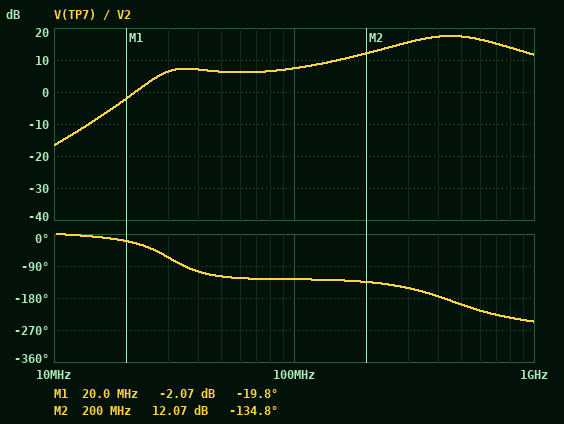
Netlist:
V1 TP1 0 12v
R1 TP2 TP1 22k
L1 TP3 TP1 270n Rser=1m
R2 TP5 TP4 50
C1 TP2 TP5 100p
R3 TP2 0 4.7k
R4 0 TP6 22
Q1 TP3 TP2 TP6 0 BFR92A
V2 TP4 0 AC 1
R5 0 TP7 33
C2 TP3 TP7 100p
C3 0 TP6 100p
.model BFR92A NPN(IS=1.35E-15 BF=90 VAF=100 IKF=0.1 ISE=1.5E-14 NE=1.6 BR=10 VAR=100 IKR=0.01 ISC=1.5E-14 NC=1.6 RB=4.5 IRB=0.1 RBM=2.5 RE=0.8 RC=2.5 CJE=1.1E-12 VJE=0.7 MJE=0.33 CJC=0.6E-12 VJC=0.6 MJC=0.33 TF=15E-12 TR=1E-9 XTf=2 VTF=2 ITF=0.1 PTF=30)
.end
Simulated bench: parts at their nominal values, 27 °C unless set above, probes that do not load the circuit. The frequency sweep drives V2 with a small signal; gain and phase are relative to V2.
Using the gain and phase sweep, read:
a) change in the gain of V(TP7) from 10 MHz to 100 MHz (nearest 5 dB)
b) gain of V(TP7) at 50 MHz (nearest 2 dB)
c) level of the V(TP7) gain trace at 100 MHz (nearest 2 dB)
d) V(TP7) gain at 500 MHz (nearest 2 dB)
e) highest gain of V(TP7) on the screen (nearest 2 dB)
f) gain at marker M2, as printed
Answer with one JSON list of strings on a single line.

["25 dB", "6 dB", "8 dB", "18 dB", "18 dB", "12.07 dB"]
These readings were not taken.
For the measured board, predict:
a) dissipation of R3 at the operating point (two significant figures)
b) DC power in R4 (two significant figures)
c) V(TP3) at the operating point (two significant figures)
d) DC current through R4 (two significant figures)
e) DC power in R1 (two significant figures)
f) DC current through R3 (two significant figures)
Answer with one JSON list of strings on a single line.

["320 µW", "8.2 mW", "12 V", "19 mA", "5.3 mW", "260 µA"]
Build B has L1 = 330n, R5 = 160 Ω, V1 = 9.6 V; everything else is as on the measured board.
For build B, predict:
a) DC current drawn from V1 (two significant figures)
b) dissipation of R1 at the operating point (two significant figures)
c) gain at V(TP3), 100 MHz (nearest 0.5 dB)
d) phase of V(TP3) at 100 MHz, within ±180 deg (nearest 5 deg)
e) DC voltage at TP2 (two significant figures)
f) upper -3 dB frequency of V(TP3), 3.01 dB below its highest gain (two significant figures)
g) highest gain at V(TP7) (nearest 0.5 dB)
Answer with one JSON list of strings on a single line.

["14 mA", "3.3 mW", "19.5 dB", "-110 deg", "1.1 V", "450 MHz", "29.5 dB"]
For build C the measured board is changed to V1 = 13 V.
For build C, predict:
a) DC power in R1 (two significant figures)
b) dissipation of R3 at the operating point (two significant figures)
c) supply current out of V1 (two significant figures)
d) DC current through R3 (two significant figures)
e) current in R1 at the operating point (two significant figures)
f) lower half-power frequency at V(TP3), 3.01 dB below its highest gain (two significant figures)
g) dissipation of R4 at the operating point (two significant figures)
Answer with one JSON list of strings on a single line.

["6.2 mW", "350 µW", "22 mA", "270 µA", "530 µA", "270 MHz", "10 mW"]
